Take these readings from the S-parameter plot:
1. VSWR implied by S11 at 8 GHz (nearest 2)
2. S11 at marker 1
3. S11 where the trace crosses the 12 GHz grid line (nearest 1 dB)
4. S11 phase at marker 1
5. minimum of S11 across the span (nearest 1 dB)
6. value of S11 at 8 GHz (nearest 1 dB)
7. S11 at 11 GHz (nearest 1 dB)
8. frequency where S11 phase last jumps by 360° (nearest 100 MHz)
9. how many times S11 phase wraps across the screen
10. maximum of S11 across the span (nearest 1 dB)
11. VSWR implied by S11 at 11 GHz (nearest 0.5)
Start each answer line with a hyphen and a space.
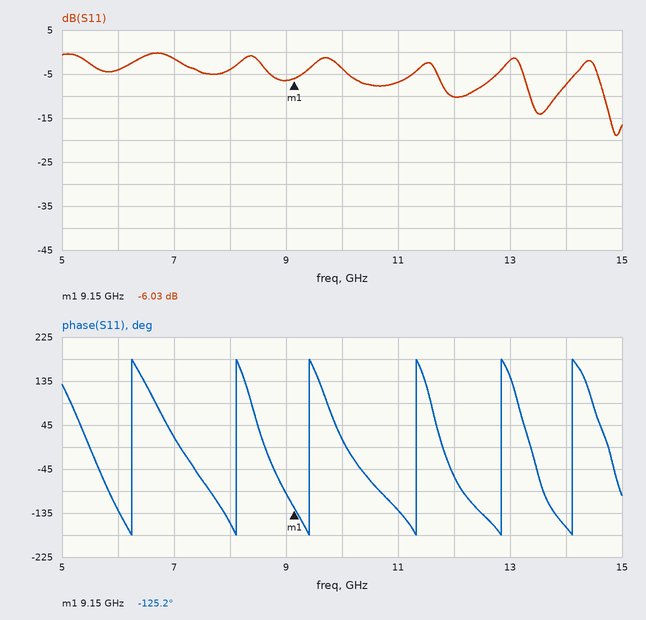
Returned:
- 4
- -6.03 dB
- -10 dB
- -125.2°
- -19 dB
- -4 dB
- -7 dB
- 14.1 GHz
- 6
- 0 dB
- 2.5
